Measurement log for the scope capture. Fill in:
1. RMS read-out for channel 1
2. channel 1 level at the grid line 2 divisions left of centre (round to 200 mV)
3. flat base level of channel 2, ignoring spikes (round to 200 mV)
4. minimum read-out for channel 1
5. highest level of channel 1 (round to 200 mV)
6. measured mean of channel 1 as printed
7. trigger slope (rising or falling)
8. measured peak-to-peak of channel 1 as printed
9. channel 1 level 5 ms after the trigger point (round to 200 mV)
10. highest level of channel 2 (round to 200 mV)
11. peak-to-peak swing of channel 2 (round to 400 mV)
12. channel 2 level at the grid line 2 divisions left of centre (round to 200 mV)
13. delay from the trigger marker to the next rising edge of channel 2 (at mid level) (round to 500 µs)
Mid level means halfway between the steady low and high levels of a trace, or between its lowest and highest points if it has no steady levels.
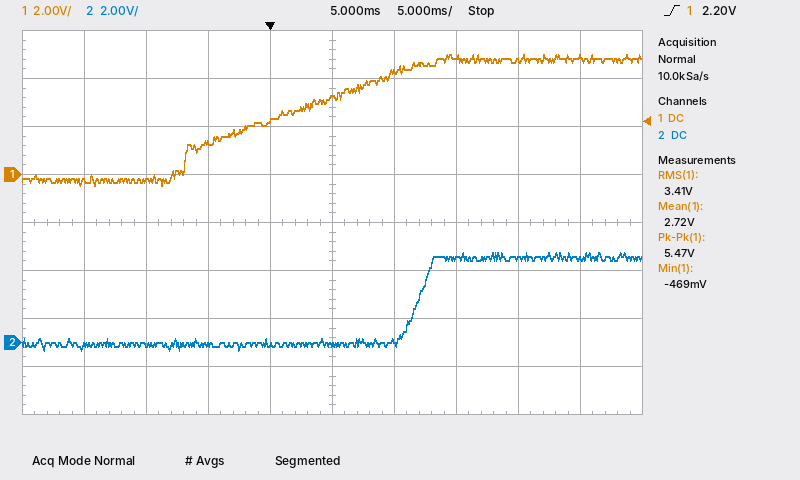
3.41 V
1.4 V
0.0 V
-469 mV
5.0 V
2.72 V
rising
5.47 V
3.2 V
3.8 V
4.0 V
0.0 V
12.0 ms
